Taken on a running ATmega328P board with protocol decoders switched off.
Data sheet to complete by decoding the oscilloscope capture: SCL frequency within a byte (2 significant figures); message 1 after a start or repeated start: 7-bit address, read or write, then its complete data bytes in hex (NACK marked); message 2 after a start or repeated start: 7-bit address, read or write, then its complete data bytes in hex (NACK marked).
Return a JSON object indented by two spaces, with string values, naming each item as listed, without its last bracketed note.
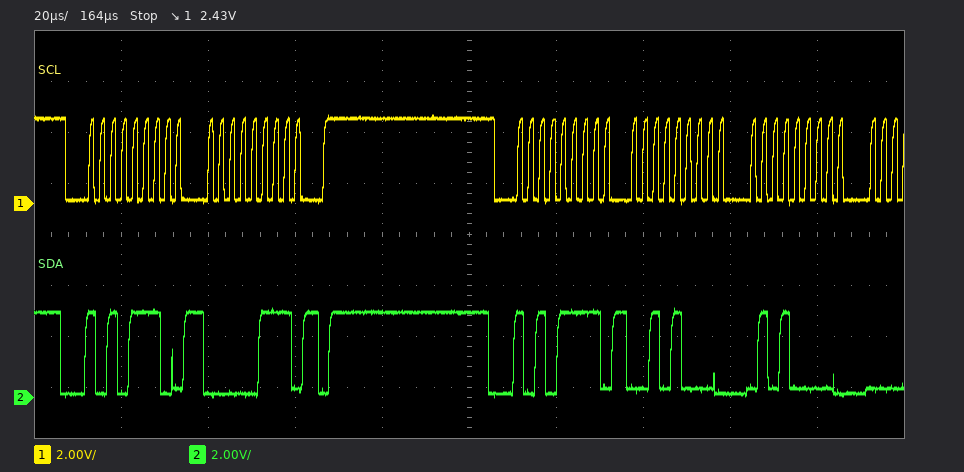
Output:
{
  "SCL frequency within a byte": "400 kHz",
  "message 1 after a start or repeated start: 7-bit address, read or write, then its complete data bytes in hex": "0x57 write: 07",
  "message 2 after a start or repeated start: 7-bit address, read or write, then its complete data bytes in hex": "0x57 read: 28 50"
}
